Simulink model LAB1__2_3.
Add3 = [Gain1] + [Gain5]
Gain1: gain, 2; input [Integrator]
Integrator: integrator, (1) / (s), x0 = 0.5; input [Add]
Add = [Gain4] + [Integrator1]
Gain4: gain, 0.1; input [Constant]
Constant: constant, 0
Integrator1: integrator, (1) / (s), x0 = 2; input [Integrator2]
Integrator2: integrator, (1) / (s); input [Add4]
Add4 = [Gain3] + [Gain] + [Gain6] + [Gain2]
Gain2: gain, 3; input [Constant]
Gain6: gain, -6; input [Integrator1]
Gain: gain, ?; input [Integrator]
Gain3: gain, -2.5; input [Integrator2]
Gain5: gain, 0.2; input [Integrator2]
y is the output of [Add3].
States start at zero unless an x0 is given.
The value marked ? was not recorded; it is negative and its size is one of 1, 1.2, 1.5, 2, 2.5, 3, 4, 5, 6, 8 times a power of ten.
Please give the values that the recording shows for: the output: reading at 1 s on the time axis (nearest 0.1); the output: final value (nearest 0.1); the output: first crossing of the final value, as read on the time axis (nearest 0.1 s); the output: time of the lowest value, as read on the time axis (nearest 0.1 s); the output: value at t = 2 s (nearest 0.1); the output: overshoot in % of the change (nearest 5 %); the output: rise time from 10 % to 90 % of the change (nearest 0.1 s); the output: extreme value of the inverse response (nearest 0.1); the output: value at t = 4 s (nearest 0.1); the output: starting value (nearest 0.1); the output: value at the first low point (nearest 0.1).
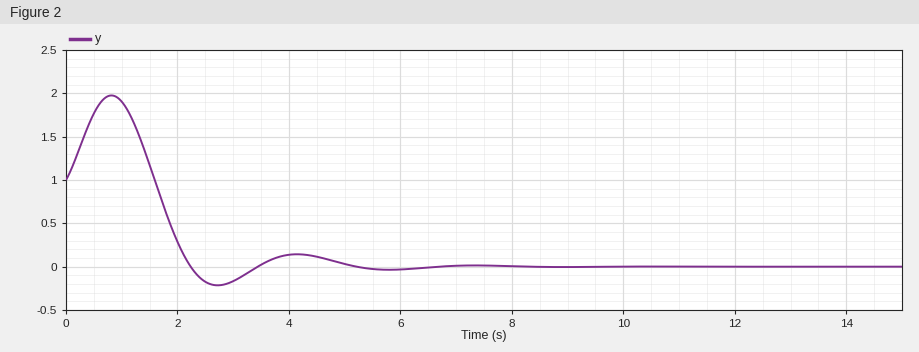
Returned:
1.9
0.0
2.2 s
2.7 s
0.3
20 %
0.5 s
2.0
0.1
1.0
-0.2
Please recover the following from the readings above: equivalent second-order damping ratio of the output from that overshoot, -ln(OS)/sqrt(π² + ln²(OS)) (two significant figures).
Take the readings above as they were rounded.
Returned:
0.46
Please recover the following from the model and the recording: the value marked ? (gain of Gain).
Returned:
-5
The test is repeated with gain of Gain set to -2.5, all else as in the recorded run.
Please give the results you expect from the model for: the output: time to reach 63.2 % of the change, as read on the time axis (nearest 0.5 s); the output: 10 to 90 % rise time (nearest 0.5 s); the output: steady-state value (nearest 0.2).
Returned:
4.5 s
4.5 s
0.0
